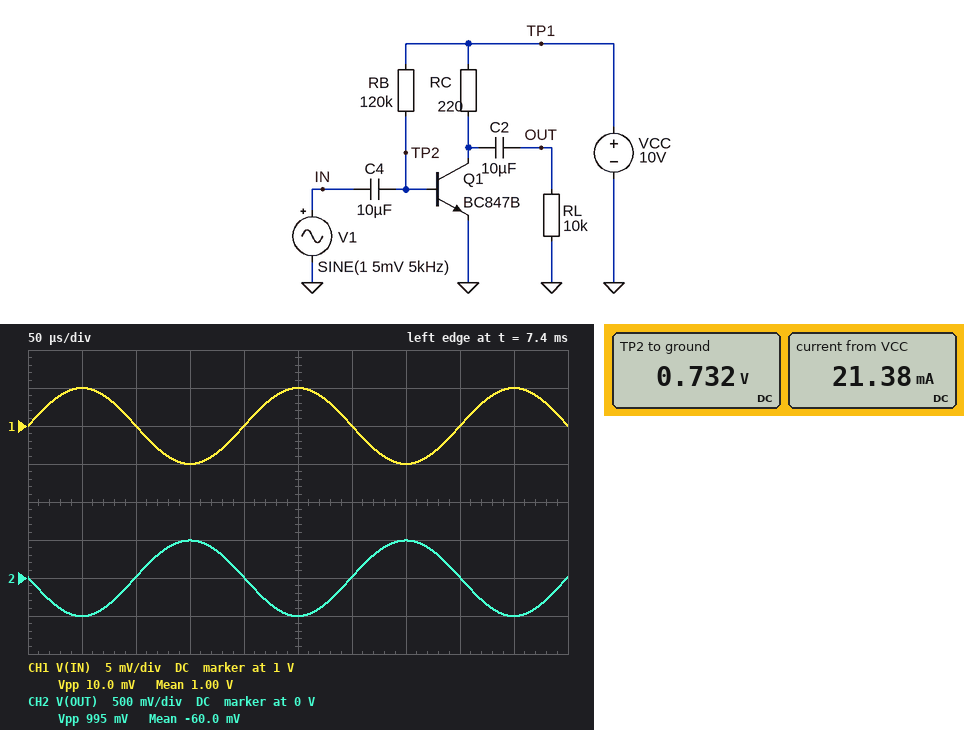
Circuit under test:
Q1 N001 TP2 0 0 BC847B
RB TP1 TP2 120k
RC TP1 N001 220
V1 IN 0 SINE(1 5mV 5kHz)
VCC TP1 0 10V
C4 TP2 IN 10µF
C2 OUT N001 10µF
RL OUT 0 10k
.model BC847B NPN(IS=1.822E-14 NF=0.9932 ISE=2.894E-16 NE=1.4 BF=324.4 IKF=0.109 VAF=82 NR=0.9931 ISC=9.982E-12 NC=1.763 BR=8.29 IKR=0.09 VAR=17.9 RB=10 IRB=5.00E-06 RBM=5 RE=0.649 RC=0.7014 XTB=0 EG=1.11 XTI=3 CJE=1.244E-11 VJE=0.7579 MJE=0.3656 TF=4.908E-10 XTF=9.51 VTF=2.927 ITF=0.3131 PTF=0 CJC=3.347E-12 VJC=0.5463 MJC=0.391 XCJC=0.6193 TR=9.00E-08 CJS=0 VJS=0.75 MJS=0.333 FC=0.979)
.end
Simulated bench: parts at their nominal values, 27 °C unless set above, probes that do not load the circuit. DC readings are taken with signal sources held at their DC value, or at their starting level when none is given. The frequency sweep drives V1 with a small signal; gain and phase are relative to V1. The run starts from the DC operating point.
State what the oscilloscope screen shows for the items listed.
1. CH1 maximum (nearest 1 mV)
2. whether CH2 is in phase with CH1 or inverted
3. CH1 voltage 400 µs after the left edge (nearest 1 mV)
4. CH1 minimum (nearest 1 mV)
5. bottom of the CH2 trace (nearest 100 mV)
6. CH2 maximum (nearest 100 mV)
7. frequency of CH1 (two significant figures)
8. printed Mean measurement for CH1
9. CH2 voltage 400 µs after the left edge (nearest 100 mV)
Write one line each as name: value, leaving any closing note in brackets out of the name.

CH1 maximum: 1.005 V
whether CH2 is in phase with CH1 or inverted: inverted
CH1 voltage 400 µs after the left edge: 1.000 V
CH1 minimum: 995 mV
bottom of the CH2 trace: -500 mV
CH2 maximum: 500 mV
frequency of CH1: 5.0 kHz
printed Mean measurement for CH1: 1.00 V
CH2 voltage 400 µs after the left edge: 0 V
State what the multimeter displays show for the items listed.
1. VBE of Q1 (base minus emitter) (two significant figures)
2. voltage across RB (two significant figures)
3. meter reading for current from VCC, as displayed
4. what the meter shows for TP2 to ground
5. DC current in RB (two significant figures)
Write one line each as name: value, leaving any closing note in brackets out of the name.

VBE of Q1 (base minus emitter): 730 mV
voltage across RB: 9.3 V
meter reading for current from VCC, as displayed: 21.38 mA
what the meter shows for TP2 to ground: 0.732 V
DC current in RB: 77 µA
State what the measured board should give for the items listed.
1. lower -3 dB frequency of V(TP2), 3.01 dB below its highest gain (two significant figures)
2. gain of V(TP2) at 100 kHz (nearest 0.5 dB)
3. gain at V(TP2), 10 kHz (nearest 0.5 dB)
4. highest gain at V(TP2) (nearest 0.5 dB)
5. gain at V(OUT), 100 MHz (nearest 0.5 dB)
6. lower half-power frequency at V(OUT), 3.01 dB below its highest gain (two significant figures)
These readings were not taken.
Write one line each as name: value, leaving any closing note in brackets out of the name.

lower -3 dB frequency of V(TP2), 3.01 dB below its highest gain: 33 Hz
gain of V(TP2) at 100 kHz: 0 dB
gain at V(TP2), 10 kHz: 0 dB
highest gain at V(TP2): 0 dB
gain at V(OUT), 100 MHz: 35.0 dB
lower half-power frequency at V(OUT), 3.01 dB below its highest gain: 33 Hz
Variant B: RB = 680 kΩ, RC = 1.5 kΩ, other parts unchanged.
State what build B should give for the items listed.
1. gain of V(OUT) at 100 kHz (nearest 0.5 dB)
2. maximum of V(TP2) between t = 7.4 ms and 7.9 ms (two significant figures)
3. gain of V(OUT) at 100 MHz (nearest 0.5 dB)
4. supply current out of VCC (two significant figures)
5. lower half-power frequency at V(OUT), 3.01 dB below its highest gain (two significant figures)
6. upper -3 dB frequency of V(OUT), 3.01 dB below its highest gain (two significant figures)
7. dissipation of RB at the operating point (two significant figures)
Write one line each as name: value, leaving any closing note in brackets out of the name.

gain of V(OUT) at 100 kHz: 45.0 dB
maximum of V(TP2) between t = 7.4 ms and 7.9 ms: 680 mV
gain of V(OUT) at 100 MHz: 37.0 dB
supply current out of VCC: 4.3 mA
lower half-power frequency at V(OUT), 3.01 dB below its highest gain: 8.0 Hz
upper -3 dB frequency of V(OUT), 3.01 dB below its highest gain: 45 MHz
dissipation of RB at the operating point: 130 µW
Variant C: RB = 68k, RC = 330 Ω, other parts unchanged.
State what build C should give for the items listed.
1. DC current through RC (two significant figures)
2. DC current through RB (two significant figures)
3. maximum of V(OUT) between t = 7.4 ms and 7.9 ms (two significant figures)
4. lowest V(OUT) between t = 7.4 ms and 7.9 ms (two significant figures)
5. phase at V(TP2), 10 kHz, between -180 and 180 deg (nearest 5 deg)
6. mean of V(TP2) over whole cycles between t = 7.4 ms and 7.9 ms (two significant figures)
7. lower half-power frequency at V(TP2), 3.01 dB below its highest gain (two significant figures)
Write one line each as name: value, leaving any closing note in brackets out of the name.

DC current through RC: 30 mA
DC current through RB: 140 µA
maximum of V(OUT) between t = 7.4 ms and 7.9 ms: 1.3 V
lowest V(OUT) between t = 7.4 ms and 7.9 ms: -100 mV
phase at V(TP2), 10 kHz, between -180 and 180 deg: 5 deg
mean of V(TP2) over whole cycles between t = 7.4 ms and 7.9 ms: 750 mV
lower half-power frequency at V(TP2), 3.01 dB below its highest gain: 610 Hz
